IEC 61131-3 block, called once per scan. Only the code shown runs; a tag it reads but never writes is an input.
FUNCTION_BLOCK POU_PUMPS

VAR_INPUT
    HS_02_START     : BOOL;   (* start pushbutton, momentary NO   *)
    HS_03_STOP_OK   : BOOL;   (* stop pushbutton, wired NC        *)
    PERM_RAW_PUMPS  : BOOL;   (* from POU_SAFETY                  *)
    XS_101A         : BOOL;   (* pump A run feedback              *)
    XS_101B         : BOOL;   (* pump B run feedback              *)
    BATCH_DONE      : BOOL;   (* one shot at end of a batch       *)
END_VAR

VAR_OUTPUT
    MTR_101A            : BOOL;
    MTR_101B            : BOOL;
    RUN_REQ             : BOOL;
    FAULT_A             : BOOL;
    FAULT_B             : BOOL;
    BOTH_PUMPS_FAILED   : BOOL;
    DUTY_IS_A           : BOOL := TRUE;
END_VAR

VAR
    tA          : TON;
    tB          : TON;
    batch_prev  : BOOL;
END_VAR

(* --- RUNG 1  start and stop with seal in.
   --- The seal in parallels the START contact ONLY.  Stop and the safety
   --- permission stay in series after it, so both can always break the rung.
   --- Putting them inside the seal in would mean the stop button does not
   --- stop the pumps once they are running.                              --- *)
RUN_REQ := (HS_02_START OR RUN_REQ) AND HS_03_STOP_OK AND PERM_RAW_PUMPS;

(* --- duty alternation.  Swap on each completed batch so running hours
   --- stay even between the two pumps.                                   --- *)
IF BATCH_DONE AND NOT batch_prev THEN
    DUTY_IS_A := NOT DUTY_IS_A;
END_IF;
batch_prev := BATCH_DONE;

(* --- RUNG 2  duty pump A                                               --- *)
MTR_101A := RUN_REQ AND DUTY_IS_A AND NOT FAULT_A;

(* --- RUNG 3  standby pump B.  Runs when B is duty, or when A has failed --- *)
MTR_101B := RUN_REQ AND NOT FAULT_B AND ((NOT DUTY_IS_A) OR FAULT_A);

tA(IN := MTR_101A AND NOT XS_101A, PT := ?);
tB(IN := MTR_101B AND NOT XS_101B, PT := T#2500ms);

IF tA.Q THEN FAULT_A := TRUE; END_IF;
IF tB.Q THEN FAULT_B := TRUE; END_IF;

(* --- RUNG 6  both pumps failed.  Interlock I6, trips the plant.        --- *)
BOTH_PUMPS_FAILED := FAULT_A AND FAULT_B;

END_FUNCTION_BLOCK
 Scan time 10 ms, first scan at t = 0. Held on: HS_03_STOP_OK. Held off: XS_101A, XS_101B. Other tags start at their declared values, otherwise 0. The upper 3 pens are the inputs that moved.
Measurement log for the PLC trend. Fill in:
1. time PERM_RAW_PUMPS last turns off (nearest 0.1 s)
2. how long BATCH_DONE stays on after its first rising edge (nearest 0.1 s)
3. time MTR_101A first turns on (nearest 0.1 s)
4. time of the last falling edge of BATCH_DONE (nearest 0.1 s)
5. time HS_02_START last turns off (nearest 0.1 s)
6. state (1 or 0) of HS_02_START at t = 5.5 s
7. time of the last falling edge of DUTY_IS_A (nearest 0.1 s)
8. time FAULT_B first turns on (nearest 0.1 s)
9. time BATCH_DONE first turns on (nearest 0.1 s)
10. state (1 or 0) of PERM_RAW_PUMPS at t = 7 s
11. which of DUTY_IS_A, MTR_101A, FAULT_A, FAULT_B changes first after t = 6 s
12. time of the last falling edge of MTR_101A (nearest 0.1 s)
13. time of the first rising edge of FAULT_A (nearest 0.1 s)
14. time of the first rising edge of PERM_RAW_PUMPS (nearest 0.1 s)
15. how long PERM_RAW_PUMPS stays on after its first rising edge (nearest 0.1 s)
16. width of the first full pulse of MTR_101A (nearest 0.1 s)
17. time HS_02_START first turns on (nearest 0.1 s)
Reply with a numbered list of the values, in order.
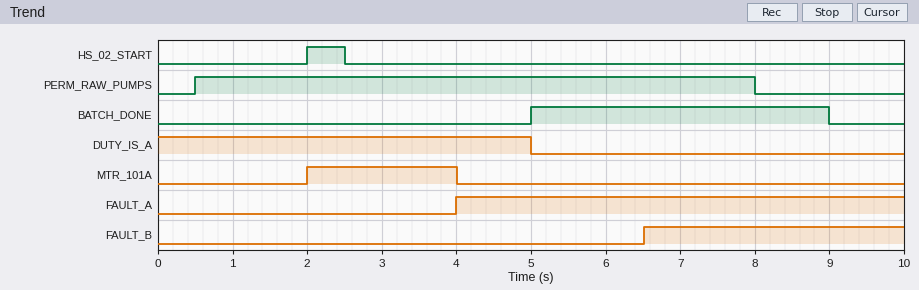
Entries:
1. 8.0 s
2. 4.0 s
3. 2.0 s
4. 9.0 s
5. 2.5 s
6. 0
7. 5.0 s
8. 6.5 s
9. 5.0 s
10. 1
11. FAULT_B
12. 4.0 s
13. 4.0 s
14. 0.5 s
15. 7.5 s
16. 2.0 s
17. 2.0 s
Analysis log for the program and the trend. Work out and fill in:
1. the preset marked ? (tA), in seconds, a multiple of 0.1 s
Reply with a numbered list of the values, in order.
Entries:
1. 2.0 s
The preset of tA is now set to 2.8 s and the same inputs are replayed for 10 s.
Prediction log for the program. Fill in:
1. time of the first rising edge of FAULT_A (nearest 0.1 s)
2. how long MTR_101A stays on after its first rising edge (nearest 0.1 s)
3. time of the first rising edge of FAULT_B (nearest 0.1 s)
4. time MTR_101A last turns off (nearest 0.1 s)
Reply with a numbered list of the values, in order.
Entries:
1. 4.8 s
2. 2.8 s
3. 7.3 s
4. 4.8 s
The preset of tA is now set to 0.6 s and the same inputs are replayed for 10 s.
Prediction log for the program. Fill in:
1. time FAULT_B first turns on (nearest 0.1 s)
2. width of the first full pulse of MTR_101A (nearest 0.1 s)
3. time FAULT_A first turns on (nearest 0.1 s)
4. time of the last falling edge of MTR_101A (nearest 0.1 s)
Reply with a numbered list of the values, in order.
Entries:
1. 5.1 s
2. 0.6 s
3. 2.6 s
4. 2.6 s
